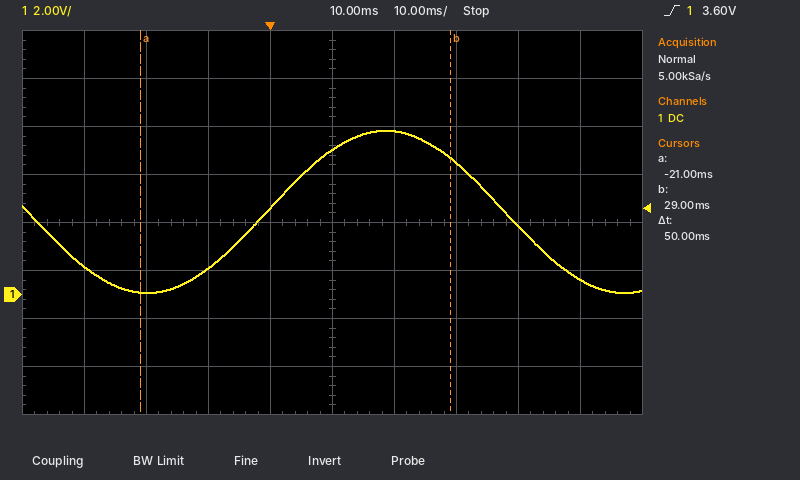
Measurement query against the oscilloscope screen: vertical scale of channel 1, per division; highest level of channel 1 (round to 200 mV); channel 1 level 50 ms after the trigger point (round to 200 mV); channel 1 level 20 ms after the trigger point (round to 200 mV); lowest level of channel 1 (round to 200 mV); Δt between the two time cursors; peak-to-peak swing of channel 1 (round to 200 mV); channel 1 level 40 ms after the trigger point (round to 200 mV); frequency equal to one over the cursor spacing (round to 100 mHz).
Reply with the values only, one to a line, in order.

2 V
6.8 V
600 mV
6.8 V
0.0 V
50 ms
6.8 V
2.8 V
20.0 Hz
